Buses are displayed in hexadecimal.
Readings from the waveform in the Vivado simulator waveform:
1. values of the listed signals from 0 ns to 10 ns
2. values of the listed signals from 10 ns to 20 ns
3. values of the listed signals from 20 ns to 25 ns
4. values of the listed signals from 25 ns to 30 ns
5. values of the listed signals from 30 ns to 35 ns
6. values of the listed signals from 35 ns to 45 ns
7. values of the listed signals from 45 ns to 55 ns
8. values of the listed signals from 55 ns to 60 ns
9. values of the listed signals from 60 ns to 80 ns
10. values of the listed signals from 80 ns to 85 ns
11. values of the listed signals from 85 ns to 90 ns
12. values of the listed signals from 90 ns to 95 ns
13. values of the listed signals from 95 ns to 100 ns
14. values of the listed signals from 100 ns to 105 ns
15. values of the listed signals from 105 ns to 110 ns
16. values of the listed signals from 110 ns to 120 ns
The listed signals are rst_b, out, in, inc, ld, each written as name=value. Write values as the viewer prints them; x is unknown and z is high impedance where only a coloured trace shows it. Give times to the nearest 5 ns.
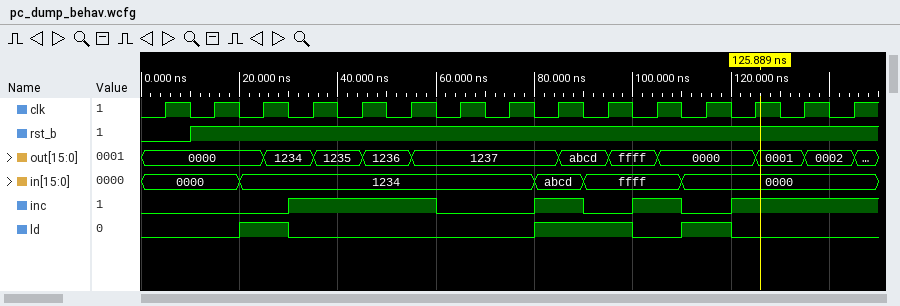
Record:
rst_b=0, out=0000, in=0000, inc=0, ld=0
rst_b=1, out=0000, in=0000, inc=0, ld=0
rst_b=1, out=0000, in=1234, inc=0, ld=1
rst_b=1, out=1234, in=1234, inc=0, ld=1
rst_b=1, out=1234, in=1234, inc=1, ld=0
rst_b=1, out=1235, in=1234, inc=1, ld=0
rst_b=1, out=1236, in=1234, inc=1, ld=0
rst_b=1, out=1237, in=1234, inc=1, ld=0
rst_b=1, out=1237, in=1234, inc=0, ld=0
rst_b=1, out=1237, in=abcd, inc=1, ld=1
rst_b=1, out=abcd, in=abcd, inc=1, ld=1
rst_b=1, out=abcd, in=ffff, inc=0, ld=1
rst_b=1, out=ffff, in=ffff, inc=0, ld=1
rst_b=1, out=ffff, in=ffff, inc=1, ld=0
rst_b=1, out=0000, in=ffff, inc=1, ld=0
rst_b=1, out=0000, in=0000, inc=0, ld=1
